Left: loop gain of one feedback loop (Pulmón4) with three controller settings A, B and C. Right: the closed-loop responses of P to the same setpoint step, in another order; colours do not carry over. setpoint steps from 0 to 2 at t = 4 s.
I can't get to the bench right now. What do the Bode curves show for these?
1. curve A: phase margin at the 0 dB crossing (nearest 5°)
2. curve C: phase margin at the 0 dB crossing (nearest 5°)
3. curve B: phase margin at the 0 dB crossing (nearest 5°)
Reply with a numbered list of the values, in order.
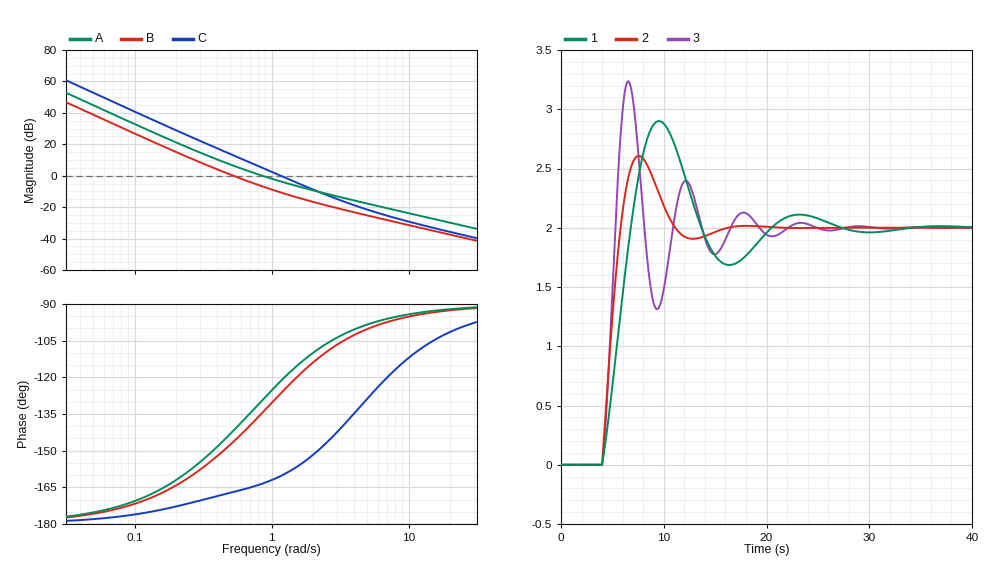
1. 50°
2. 20°
3. 35°
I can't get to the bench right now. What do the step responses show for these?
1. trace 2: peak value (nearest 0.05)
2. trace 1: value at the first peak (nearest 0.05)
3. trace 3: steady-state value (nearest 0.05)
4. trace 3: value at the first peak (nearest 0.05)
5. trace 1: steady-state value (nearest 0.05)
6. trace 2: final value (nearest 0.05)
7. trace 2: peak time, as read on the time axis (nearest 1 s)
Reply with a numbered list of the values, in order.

1. 2.60
2. 2.90
3. 2.00
4. 3.25
5. 2.00
6. 2.00
7. 8 s
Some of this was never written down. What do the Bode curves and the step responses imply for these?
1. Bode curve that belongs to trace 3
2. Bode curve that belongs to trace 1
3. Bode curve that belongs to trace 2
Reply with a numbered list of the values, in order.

1. C
2. B
3. A
